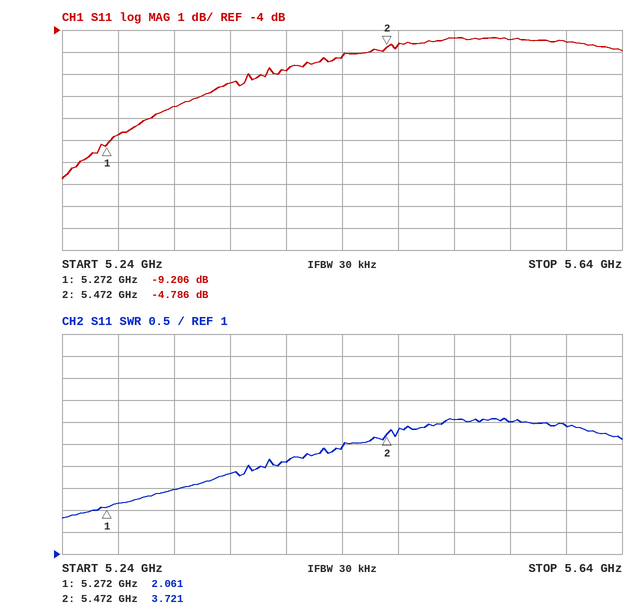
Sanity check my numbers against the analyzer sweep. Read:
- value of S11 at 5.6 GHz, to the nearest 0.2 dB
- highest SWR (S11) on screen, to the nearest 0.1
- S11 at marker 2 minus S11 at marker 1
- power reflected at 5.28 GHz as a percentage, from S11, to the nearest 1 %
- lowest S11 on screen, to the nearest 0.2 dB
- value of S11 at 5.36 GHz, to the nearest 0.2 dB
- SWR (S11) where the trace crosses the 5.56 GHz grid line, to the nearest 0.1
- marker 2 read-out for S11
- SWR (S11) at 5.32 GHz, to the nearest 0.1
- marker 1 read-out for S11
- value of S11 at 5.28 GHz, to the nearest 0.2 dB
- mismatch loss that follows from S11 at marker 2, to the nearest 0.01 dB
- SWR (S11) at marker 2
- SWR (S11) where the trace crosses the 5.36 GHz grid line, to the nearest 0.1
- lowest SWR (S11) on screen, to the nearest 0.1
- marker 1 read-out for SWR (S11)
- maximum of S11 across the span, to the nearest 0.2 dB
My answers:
-4.6 dB
4.1
4.420 dB
13 %
-10.8 dB
-6.4 dB
4.0
-4.786 dB
2.5
-9.206 dB
-8.8 dB
1.75 dB
3.721
2.8
1.8
2.061
-4.4 dB
